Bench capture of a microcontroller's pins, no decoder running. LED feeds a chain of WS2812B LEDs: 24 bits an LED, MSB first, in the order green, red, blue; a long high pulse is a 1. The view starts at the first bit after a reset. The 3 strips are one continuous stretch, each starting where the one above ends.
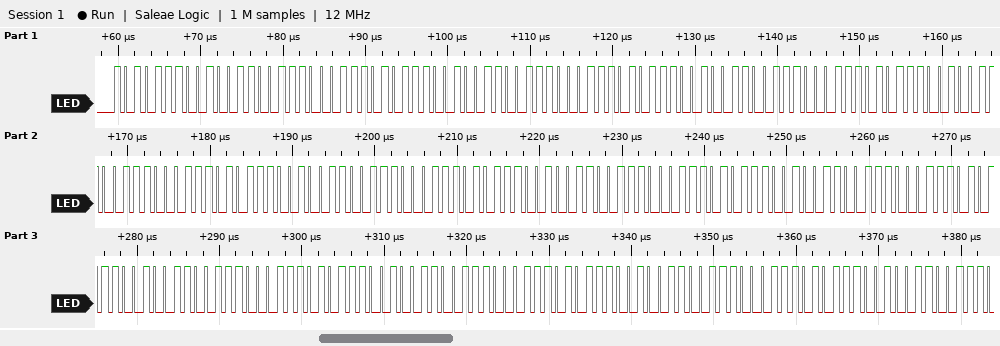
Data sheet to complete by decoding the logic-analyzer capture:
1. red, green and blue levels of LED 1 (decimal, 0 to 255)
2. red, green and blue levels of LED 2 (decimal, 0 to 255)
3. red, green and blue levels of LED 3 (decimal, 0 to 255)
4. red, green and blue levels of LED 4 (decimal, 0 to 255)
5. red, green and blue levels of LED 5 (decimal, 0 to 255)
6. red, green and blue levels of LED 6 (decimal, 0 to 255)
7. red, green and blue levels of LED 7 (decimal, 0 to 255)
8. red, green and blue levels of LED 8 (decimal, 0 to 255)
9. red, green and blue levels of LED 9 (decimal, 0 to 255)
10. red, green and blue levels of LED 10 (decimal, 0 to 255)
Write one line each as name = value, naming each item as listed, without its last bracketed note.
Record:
red, green and blue levels of LED 1 = 76, 174, 227
red, green and blue levels of LED 2 = 76, 174, 227
red, green and blue levels of LED 3 = 76, 174, 227
red, green and blue levels of LED 4 = 76, 174, 227
red, green and blue levels of LED 5 = 76, 174, 227
red, green and blue levels of LED 6 = 76, 174, 227
red, green and blue levels of LED 7 = 76, 174, 227
red, green and blue levels of LED 8 = 76, 174, 227
red, green and blue levels of LED 9 = 76, 174, 227
red, green and blue levels of LED 10 = 76, 174, 227
